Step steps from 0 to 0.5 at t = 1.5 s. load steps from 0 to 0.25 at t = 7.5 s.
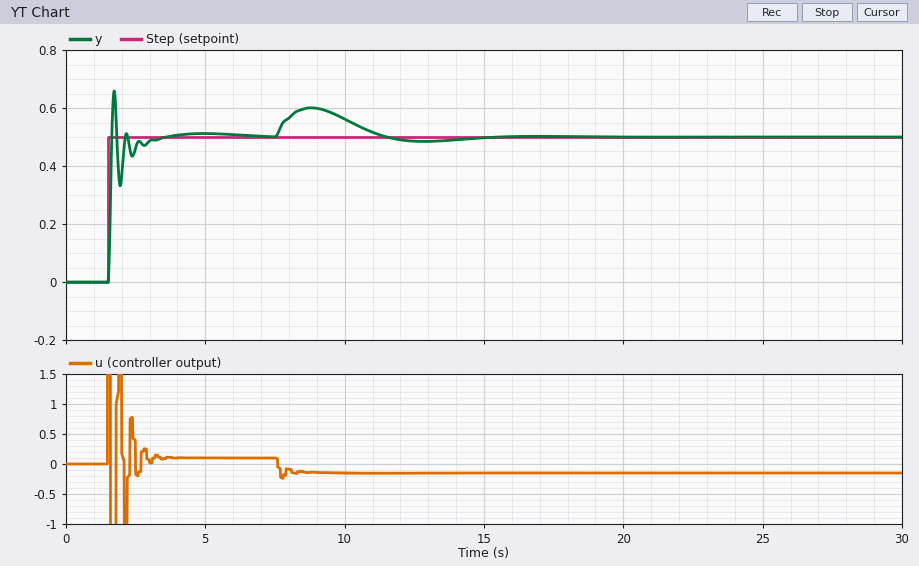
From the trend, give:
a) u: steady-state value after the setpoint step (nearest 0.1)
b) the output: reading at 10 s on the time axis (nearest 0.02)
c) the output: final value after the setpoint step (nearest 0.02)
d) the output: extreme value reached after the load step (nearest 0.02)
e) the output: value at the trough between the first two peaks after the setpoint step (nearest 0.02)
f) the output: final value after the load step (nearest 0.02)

0.1
0.56
0.50
0.60
0.34
0.50
